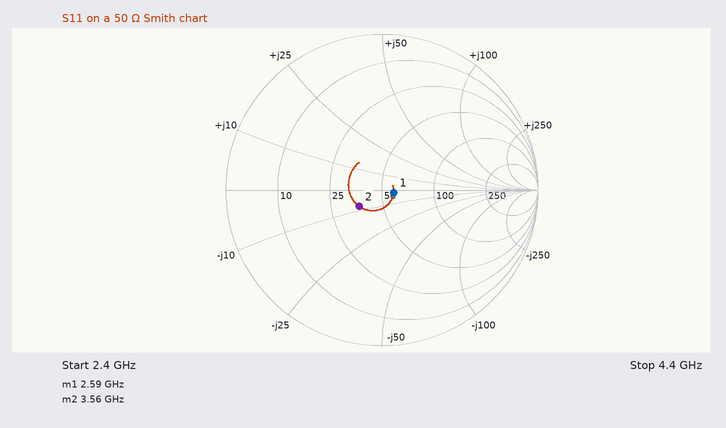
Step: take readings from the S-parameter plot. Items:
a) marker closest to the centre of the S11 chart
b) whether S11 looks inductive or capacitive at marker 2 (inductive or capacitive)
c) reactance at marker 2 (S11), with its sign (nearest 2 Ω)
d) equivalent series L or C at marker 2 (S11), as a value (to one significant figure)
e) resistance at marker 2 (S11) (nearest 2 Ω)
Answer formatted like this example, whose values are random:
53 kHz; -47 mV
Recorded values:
marker 1; capacitive; -8 Ω; 6 pF; 36 Ω
